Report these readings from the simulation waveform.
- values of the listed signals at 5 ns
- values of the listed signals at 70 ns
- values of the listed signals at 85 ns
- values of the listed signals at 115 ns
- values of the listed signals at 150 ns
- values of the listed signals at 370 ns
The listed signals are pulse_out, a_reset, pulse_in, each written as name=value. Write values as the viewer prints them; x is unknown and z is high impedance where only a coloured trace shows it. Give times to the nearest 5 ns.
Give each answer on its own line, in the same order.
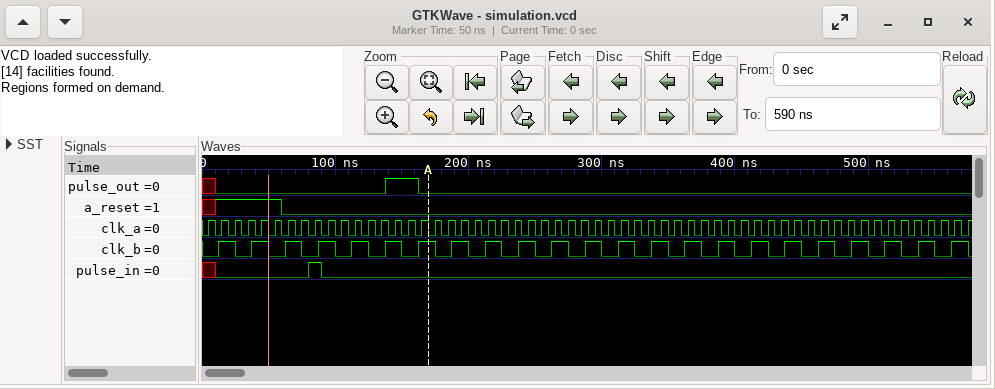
pulse_out=x, a_reset=x, pulse_in=x
pulse_out=0, a_reset=0, pulse_in=0
pulse_out=0, a_reset=0, pulse_in=1
pulse_out=0, a_reset=0, pulse_in=0
pulse_out=1, a_reset=0, pulse_in=0
pulse_out=0, a_reset=0, pulse_in=0
